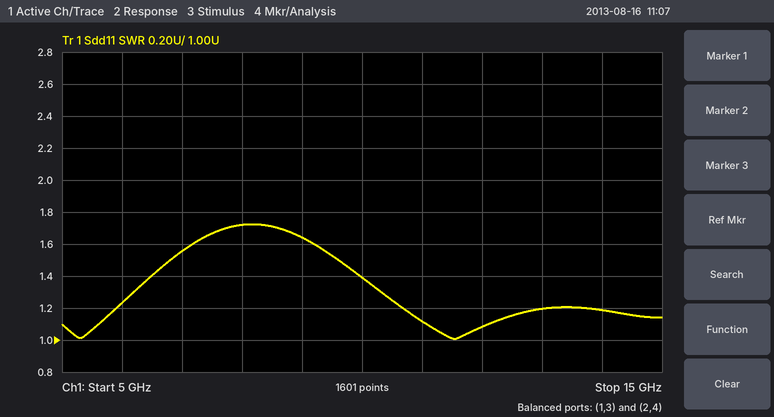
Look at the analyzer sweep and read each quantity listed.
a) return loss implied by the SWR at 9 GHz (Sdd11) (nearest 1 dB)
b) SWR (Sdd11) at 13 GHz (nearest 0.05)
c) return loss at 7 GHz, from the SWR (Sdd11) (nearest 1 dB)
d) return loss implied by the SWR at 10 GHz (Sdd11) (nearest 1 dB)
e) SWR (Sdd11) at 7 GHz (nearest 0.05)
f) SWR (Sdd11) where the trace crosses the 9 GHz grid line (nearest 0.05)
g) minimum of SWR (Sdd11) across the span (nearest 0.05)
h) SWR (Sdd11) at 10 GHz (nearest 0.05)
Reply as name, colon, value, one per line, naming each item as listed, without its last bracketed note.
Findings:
return loss implied by the SWR at 9 GHz (Sdd11): 12 dB
SWR (Sdd11) at 13 GHz: 1.20
return loss at 7 GHz, from the SWR (Sdd11): 13 dB
return loss implied by the SWR at 10 GHz (Sdd11): 16 dB
SWR (Sdd11) at 7 GHz: 1.55
SWR (Sdd11) where the trace crosses the 9 GHz grid line: 1.65
minimum of SWR (Sdd11) across the span: 1.00
SWR (Sdd11) at 10 GHz: 1.40
